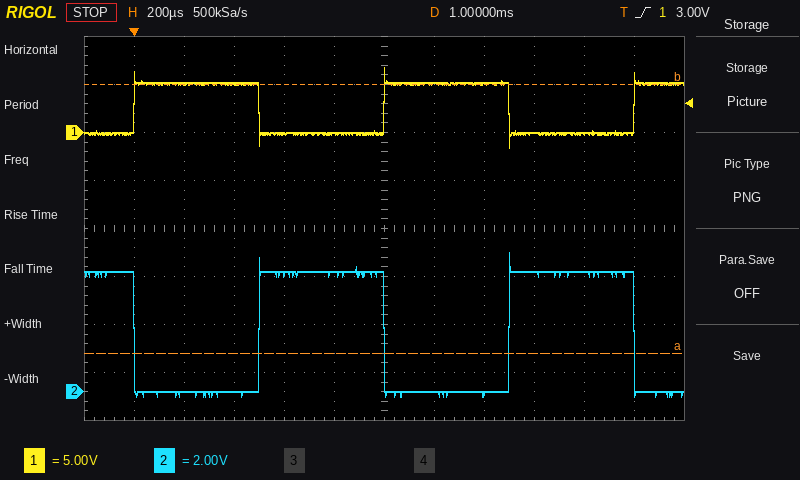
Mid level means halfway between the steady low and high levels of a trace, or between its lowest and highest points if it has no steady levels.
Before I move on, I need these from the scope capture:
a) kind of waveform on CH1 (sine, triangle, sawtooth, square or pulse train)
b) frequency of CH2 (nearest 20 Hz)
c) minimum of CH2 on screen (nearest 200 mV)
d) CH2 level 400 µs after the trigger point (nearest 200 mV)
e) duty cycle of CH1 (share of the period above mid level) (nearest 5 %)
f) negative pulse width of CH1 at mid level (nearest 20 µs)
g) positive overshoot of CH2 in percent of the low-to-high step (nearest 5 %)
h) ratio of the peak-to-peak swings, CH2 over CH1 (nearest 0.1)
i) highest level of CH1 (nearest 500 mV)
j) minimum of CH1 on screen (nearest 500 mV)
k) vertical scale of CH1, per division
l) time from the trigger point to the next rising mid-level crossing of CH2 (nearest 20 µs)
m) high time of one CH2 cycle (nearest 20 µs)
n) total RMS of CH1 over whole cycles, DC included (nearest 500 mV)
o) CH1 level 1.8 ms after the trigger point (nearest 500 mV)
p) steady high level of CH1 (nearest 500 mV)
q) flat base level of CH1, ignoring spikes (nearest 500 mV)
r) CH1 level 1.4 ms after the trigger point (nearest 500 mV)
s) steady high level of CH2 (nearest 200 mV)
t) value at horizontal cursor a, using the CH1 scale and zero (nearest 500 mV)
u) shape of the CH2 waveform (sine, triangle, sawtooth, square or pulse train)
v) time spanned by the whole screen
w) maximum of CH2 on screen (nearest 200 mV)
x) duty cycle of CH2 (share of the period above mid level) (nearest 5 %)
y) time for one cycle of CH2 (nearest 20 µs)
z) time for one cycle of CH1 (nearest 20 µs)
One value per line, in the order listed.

square
1.00 kHz
-200 mV
0.0 V
50 %
500 µs
15 %
0.7
7.0 V
-1.5 V
5 V
500 µs
500 µs
3.5 V
0.0 V
5.0 V
0.0 V
5.0 V
5.0 V
-23.0 V
square
2.4 ms
5.8 V
50 %
1.00 ms
1.00 ms
